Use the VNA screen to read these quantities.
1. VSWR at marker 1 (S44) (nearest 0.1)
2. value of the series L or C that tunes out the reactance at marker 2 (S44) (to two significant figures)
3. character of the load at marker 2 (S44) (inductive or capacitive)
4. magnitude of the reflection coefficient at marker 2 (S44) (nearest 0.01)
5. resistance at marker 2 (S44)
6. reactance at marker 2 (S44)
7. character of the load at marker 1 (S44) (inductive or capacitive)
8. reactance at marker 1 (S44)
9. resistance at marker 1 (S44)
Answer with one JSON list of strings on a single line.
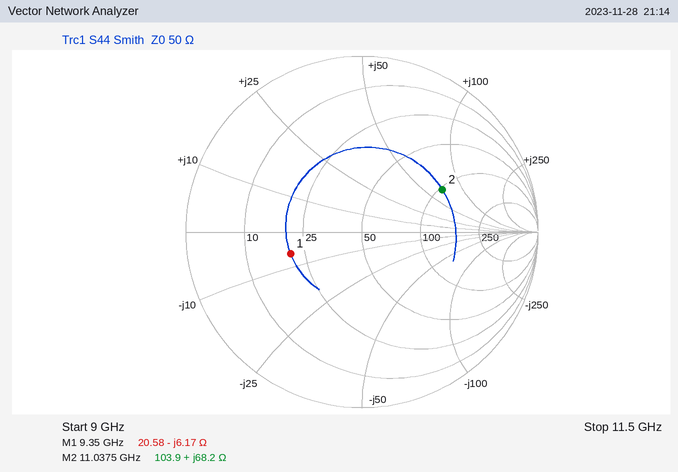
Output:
["2.5", "210 fF", "inductive", "0.52", "103.9 Ω", "+68.2 Ω", "capacitive", "-6.17 Ω", "20.58 Ω"]
